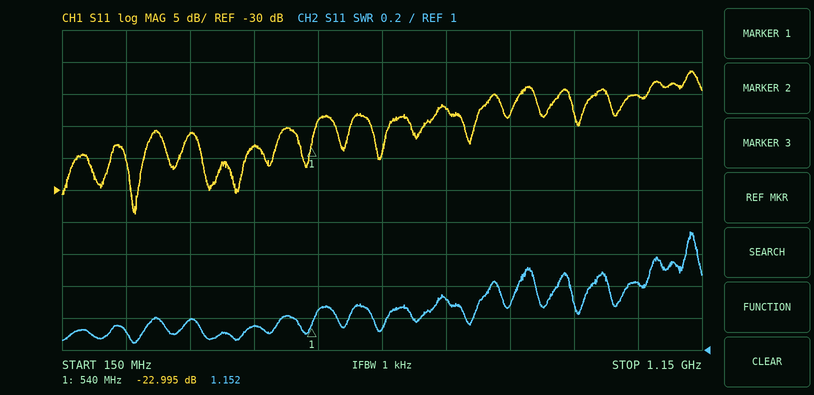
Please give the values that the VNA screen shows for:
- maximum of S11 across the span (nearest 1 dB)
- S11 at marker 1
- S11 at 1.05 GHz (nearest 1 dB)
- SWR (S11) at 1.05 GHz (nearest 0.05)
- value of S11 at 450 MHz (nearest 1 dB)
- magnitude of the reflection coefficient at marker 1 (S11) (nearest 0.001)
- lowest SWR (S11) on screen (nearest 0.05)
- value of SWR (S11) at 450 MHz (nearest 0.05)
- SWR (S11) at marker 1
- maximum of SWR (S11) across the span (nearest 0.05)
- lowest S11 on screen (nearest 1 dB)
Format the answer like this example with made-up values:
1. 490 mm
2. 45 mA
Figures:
1. -11 dB
2. -22.995 dB
3. -15 dB
4. 1.40
5. -23 dB
6. 0.071
7. 1.05
8. 1.15
9. 1.152
10. 1.75
11. -34 dB
